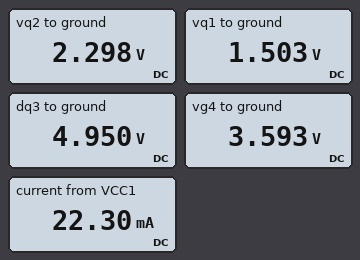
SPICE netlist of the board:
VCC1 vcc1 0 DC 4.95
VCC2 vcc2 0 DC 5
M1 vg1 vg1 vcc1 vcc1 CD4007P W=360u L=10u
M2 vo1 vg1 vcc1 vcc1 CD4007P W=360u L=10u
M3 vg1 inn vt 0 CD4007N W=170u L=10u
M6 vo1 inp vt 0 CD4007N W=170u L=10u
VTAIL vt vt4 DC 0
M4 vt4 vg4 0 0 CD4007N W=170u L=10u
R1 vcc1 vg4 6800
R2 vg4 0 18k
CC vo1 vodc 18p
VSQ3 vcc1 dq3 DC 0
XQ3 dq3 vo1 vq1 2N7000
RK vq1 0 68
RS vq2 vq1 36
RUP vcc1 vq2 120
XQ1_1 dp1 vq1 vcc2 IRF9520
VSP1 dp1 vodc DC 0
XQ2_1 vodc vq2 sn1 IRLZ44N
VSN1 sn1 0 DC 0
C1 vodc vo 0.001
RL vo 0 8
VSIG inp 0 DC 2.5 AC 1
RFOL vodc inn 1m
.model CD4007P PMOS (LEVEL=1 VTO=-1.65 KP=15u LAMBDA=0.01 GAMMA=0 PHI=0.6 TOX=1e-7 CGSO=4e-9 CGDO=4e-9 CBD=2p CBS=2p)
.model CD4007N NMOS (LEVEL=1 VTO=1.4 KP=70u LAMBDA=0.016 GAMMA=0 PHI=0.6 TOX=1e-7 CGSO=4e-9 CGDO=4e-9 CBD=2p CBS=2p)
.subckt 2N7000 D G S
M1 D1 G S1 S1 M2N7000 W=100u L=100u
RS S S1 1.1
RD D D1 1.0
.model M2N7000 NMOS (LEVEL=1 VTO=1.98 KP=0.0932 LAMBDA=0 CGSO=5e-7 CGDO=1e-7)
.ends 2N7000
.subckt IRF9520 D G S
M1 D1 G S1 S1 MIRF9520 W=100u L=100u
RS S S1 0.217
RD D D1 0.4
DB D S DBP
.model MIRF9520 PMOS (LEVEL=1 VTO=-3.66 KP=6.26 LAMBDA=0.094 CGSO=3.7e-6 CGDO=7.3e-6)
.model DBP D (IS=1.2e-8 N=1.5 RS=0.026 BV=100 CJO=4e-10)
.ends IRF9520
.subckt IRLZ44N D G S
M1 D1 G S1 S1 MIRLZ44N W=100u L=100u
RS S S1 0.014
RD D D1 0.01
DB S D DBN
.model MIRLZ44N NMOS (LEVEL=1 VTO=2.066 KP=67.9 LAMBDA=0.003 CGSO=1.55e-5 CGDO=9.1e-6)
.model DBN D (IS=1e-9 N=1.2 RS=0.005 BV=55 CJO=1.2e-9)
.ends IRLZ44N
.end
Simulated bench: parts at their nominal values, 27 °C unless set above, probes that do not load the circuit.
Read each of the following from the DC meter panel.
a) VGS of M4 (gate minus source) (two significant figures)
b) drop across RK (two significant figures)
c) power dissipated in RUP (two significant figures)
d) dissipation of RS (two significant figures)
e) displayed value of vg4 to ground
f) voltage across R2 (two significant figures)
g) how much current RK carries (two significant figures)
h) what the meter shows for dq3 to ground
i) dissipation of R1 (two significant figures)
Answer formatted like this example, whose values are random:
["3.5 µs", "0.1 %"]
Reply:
["3.6 V", "1.5 V", "59 mW", "18 mW", "3.593 V", "3.6 V", "22 mA", "4.950 V", "270 µW"]
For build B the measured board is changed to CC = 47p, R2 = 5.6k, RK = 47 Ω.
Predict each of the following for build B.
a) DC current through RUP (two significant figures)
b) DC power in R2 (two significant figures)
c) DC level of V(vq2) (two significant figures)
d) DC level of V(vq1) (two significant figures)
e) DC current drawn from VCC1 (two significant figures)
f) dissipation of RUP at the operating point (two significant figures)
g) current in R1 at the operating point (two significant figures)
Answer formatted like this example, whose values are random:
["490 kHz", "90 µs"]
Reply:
["24 mA", "890 µW", "2.1 V", "1.2 V", "27 mA", "68 mW", "400 µA"]
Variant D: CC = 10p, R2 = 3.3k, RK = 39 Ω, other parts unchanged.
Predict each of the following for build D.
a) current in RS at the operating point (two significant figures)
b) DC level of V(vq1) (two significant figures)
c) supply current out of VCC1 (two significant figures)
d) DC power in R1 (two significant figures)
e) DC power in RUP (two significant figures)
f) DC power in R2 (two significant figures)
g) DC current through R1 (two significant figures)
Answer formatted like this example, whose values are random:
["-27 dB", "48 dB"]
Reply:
["24 mA", "1.2 V", "32 mA", "1.6 mW", "68 mW", "790 µW", "490 µA"]
